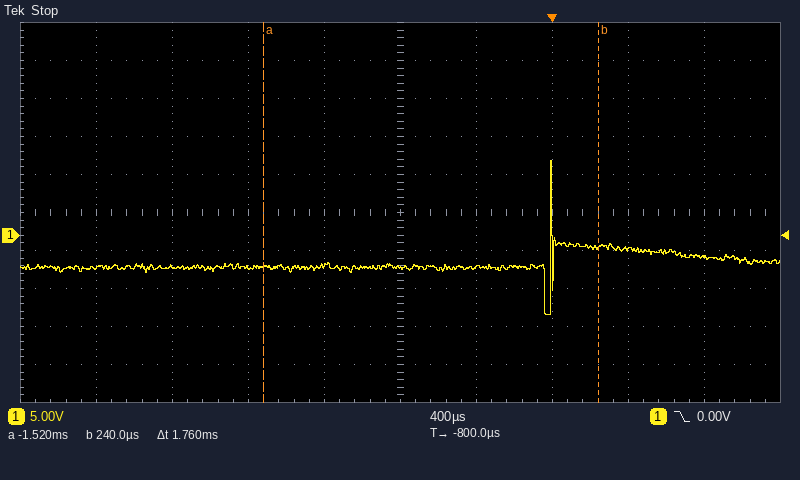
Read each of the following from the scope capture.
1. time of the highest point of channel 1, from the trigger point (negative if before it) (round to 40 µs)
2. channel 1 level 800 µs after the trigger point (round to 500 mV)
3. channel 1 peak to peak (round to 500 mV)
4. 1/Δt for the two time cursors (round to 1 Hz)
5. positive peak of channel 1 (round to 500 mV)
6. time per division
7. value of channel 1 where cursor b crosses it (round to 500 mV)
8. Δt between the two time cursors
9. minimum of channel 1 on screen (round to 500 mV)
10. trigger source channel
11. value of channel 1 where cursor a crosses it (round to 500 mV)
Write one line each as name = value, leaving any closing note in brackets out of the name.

time of the highest point of channel 1, from the trigger point (negative if before it) = 0 µs
channel 1 level 800 µs after the trigger point = -3.0 V
channel 1 peak to peak = 20.5 V
1/Δt for the two time cursors = 568 Hz
positive peak of channel 1 = 10.0 V
time per division = 400 µs
value of channel 1 where cursor b crosses it = -1.5 V
Δt between the two time cursors = 1.76 ms
minimum of channel 1 on screen = -10.5 V
trigger source channel = channel 1
value of channel 1 where cursor a crosses it = -4.0 V
